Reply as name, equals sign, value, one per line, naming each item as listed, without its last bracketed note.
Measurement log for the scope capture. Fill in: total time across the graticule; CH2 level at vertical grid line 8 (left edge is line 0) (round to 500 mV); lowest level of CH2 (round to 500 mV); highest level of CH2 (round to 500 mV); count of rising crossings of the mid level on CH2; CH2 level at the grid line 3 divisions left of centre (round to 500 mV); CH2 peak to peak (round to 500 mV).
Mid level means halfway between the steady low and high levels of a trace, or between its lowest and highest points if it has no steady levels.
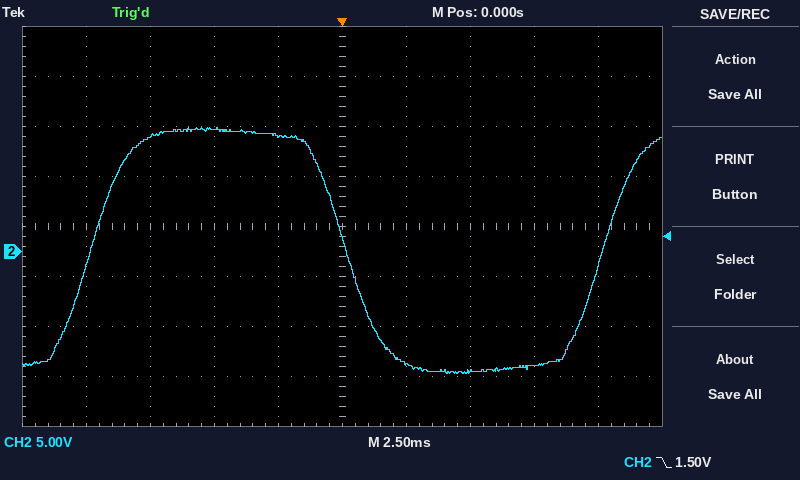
total time across the graticule = 25 ms
CH2 level at vertical grid line 8 (left edge is line 0) = -11.5 V
lowest level of CH2 = -12.0 V
highest level of CH2 = 12.5 V
count of rising crossings of the mid level on CH2 = 2
CH2 level at the grid line 3 divisions left of centre = 11.5 V
CH2 peak to peak = 24.5 V
